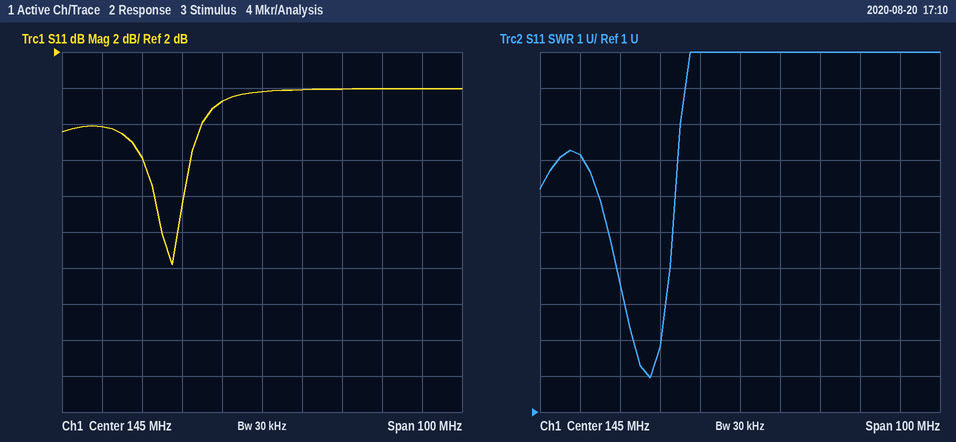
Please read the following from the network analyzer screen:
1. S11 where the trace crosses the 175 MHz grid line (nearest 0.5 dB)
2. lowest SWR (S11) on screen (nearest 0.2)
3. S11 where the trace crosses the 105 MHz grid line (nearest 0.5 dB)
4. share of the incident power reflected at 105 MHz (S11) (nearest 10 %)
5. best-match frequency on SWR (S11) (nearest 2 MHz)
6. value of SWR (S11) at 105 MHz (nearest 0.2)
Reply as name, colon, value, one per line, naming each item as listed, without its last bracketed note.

S11 where the trace crosses the 175 MHz grid line: 0.0 dB
lowest SWR (S11) on screen: 2.0
S11 where the trace crosses the 105 MHz grid line: -2.0 dB
share of the incident power reflected at 105 MHz (S11): 60 %
best-match frequency on SWR (S11): 122 MHz
value of SWR (S11) at 105 MHz: 8.2
